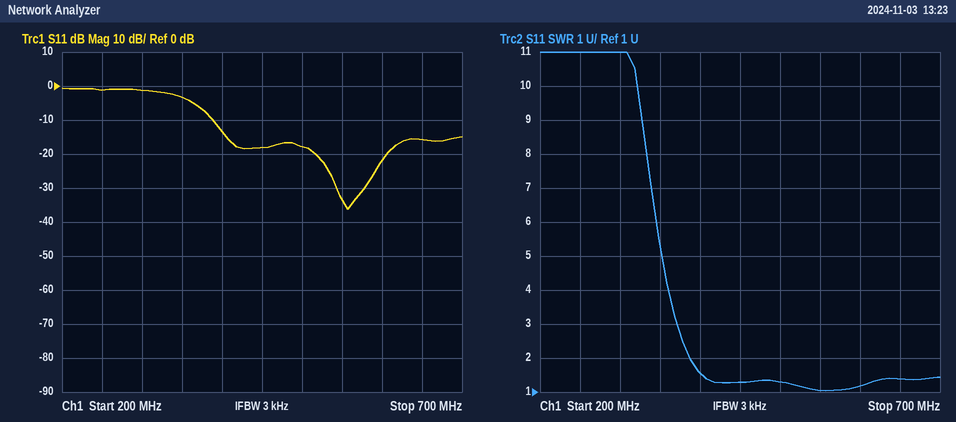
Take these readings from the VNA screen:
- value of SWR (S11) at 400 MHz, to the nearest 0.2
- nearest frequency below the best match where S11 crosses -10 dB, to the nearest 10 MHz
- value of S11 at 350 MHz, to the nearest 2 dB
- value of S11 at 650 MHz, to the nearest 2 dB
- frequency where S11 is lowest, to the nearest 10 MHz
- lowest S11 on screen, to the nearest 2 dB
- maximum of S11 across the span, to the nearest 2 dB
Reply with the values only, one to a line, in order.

1.6
390 MHz
-4 dB
-16 dB
560 MHz
-36 dB
0 dB
